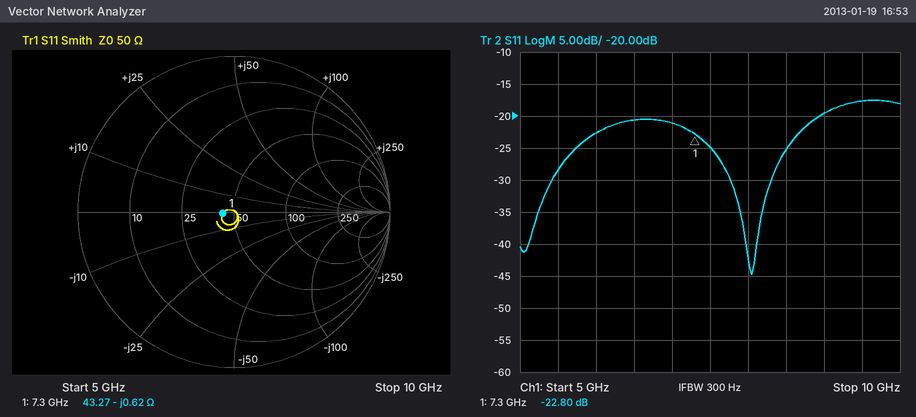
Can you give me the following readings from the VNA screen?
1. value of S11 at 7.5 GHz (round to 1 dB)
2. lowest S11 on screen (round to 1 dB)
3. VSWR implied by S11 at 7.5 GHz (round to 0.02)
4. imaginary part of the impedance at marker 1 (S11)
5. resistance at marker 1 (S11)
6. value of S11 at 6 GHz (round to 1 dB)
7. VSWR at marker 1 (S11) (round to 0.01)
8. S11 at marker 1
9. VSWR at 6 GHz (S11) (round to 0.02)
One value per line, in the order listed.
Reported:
-25 dB
-45 dB
1.12
-0.62 Ω
43.27 Ω
-23 dB
1.16
-22.80 dB
1.16
